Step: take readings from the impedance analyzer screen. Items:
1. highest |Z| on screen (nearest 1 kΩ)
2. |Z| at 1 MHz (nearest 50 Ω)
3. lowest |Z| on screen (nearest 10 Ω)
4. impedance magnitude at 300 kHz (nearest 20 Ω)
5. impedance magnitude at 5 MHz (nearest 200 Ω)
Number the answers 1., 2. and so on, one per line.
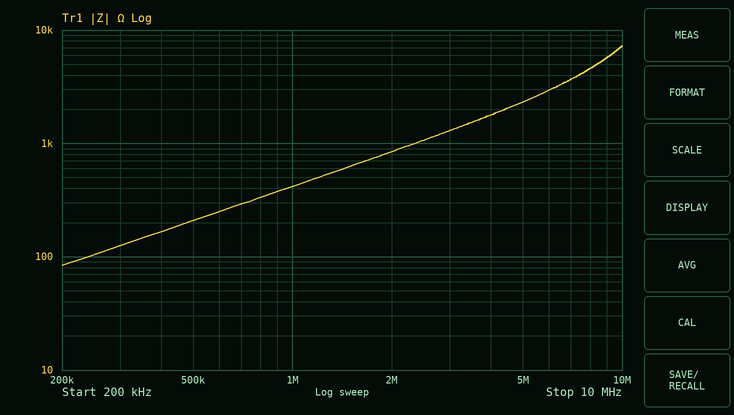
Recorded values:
1. 7 kΩ
2. 400 Ω
3. 80 Ω
4. 120 Ω
5. 2.4 kΩ
